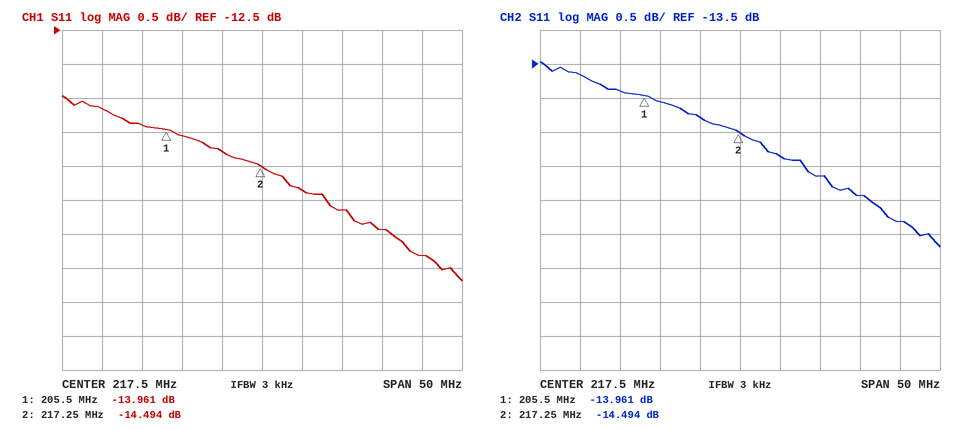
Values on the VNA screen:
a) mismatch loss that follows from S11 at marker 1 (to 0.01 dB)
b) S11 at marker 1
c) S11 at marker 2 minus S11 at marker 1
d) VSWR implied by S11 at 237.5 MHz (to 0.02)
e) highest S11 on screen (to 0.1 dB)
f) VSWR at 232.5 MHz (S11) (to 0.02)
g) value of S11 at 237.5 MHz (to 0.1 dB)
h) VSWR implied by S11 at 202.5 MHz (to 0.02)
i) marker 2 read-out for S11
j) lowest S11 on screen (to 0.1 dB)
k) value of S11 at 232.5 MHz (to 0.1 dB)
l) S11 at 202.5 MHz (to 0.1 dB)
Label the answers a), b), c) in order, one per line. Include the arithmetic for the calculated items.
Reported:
a) −10 log10(1 − 10^(-13.961/10)) ≈ 0.18 dB
b) -13.961 dB
c) -14.494 − (-13.961) = -0.533 dB
d) |Γ| = 10^(-15.8/20) = 0.1622; VSWR = (1 + 0.1622)/(1 − 0.1622) ≈ 1.39, so 1.38 to the nearest 0.02
e) -13.5 dB
f) |Γ| = 10^(-15.4/20) = 0.1698; VSWR = (1 + 0.1698)/(1 − 0.1698) ≈ 1.41, so 1.40 to the nearest 0.02
g) -15.8 dB
h) |Γ| = 10^(-13.9/20) = 0.2018; VSWR = (1 + 0.2018)/(1 − 0.2018) ≈ 1.51, so 1.50 to the nearest 0.02
i) -14.494 dB
j) -16.2 dB
k) -15.4 dB
l) -13.9 dB
